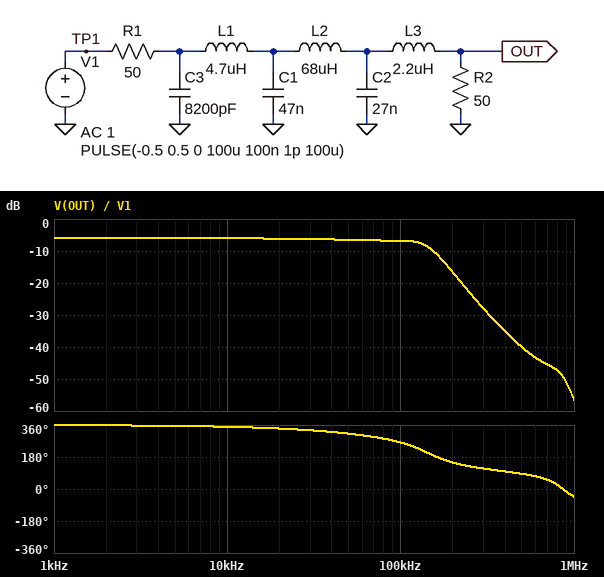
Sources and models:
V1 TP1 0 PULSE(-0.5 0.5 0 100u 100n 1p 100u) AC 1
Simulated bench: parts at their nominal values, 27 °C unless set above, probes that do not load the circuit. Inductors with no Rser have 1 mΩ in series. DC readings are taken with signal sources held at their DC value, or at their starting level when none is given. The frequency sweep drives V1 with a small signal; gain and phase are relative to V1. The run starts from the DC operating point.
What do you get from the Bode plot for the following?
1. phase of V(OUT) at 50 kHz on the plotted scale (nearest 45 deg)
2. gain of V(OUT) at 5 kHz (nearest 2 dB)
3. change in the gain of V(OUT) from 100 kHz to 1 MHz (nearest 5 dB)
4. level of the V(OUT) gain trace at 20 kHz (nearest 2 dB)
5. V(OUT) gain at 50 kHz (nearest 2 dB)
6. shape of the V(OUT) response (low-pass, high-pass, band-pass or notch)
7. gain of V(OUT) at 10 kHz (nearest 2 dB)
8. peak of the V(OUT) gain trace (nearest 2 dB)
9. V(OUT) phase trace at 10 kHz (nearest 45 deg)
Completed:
315 deg
-6 dB
-50 dB
-6 dB
-6 dB
low-pass
-6 dB
-6 dB
360 deg
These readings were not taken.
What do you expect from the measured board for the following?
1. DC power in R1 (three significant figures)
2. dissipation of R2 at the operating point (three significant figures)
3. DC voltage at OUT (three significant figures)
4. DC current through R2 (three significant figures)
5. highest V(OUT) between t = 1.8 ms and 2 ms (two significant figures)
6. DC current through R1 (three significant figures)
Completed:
1.25 mW
1.25 mW
-250 mV
5.00 mA
240 mV
5.00 mA
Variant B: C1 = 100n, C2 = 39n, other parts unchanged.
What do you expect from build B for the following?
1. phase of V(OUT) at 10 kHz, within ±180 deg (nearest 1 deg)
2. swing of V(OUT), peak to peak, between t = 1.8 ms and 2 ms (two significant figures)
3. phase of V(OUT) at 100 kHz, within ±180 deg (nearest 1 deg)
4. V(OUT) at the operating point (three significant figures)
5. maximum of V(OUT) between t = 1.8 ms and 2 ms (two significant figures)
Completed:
-16 deg
450 mV
-138 deg
-250 mV
230 mV
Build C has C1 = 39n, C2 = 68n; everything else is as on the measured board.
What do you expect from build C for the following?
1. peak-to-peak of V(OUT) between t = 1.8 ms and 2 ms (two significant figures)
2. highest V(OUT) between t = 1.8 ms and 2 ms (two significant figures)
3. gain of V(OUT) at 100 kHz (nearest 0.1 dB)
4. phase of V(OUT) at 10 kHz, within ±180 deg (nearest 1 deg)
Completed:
490 mV
230 mV
-6.4 dB
-13 deg
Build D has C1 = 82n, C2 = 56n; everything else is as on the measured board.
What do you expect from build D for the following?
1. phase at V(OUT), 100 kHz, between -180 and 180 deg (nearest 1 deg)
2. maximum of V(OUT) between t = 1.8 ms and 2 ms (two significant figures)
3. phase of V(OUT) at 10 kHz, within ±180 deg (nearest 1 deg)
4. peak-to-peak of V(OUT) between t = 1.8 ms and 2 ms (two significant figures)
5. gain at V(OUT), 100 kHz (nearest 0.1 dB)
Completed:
-151 deg
230 mV
-16 deg
470 mV
-7.0 dB
